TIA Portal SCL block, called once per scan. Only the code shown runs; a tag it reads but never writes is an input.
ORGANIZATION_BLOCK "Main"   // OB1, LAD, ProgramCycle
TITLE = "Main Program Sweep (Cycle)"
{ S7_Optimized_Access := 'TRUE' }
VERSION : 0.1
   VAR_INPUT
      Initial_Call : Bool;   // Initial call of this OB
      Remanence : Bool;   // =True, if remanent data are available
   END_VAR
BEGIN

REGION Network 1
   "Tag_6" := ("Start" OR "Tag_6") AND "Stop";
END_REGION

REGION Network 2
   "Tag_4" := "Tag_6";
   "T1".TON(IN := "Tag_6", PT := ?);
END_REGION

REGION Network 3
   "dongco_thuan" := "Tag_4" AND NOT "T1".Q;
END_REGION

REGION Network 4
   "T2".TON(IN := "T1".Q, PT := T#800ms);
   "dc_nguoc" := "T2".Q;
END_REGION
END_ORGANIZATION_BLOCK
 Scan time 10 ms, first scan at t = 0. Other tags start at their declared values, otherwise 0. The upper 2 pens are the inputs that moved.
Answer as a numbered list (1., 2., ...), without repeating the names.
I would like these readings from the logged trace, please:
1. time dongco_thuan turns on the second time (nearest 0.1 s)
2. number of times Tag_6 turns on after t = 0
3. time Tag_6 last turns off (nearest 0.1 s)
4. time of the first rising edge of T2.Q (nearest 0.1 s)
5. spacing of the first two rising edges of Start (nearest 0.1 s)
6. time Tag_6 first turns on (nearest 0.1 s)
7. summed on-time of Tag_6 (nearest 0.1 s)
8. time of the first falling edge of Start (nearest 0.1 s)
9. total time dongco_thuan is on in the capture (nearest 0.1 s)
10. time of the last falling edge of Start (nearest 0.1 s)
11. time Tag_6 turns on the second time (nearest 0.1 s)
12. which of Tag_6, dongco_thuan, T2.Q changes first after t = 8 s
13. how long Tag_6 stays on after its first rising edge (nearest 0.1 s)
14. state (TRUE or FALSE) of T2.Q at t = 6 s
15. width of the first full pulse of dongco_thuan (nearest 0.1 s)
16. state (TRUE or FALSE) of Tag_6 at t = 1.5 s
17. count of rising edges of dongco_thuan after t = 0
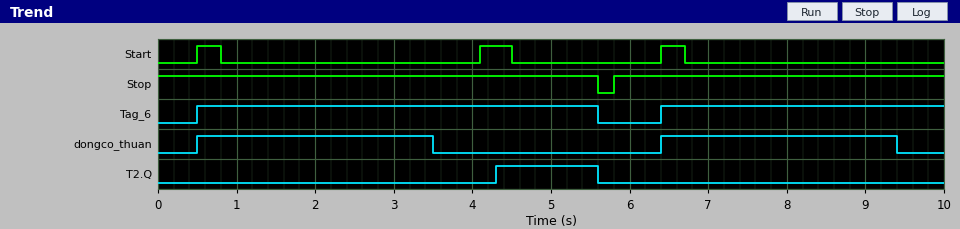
1. 6.4 s
2. 2
3. 5.6 s
4. 4.3 s
5. 3.6 s
6. 0.5 s
7. 8.7 s
8. 0.8 s
9. 6.0 s
10. 6.7 s
11. 6.4 s
12. dongco_thuan
13. 5.1 s
14. FALSE
15. 3.0 s
16. TRUE
17. 2
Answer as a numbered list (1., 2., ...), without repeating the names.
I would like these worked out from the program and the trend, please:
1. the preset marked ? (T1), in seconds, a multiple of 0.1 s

1. 3.0 s
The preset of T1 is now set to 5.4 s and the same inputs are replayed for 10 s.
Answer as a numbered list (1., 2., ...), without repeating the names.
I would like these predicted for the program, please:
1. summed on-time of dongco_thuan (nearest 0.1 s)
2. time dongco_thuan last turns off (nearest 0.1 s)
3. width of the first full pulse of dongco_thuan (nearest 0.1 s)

1. 8.7 s
2. 5.6 s
3. 5.1 s
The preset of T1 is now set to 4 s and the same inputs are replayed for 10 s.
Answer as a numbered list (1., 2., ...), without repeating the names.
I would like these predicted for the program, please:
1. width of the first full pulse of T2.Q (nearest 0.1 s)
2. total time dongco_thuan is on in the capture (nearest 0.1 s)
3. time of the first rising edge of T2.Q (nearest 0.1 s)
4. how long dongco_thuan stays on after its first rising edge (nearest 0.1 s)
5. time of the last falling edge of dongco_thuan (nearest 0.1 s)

1. 0.3 s
2. 7.6 s
3. 5.3 s
4. 4.0 s
5. 4.5 s
